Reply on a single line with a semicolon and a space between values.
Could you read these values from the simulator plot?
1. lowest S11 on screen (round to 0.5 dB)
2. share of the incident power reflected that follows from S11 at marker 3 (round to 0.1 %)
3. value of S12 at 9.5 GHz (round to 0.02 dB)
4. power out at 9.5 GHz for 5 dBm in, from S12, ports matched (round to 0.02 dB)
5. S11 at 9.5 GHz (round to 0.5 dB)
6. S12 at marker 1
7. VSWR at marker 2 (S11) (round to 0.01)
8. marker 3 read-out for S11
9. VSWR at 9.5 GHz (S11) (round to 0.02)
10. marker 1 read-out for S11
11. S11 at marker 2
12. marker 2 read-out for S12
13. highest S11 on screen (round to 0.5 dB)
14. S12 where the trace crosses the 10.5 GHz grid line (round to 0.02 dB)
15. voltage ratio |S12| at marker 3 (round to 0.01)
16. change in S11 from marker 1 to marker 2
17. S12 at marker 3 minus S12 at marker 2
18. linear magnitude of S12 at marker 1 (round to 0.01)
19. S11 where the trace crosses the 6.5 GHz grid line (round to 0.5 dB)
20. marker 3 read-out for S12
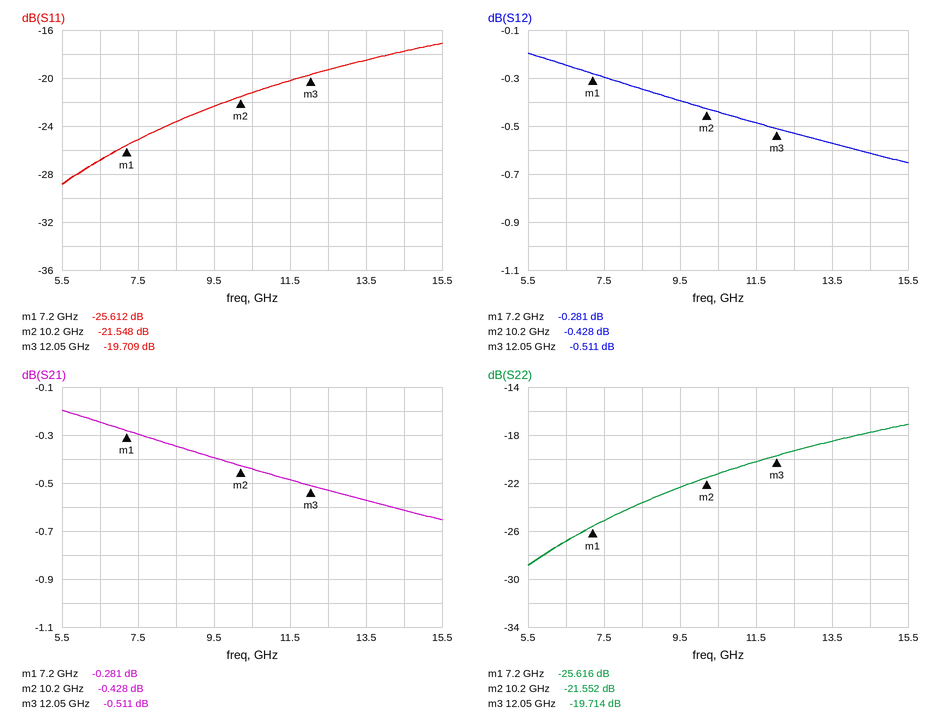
-29.0 dB; 1.1 %; -0.40 dB; 4.60 dBm; -22.5 dB; -0.281 dB; 1.18; -19.709 dB; 1.16; -25.612 dB; -21.548 dB; -0.428 dB; -17.0 dB; -0.44 dB; 0.94; 4.064 dB; -0.083 dB; 0.97; -27.0 dB; -0.511 dB
